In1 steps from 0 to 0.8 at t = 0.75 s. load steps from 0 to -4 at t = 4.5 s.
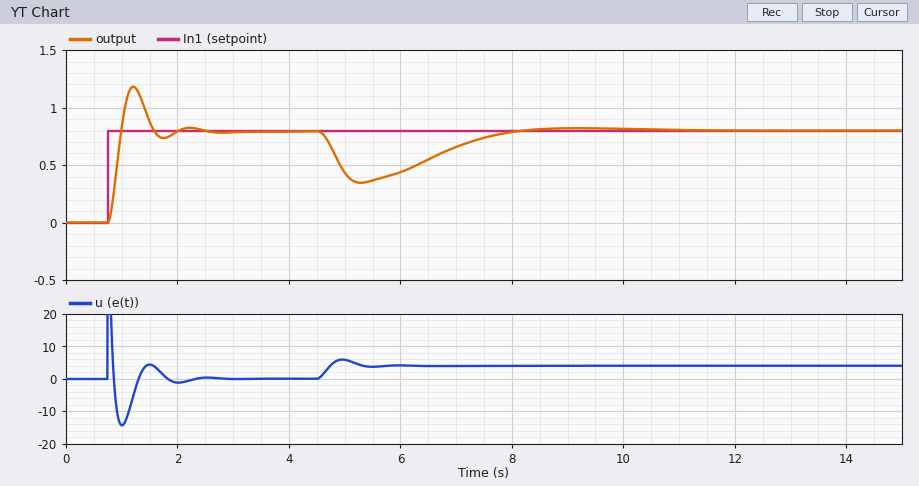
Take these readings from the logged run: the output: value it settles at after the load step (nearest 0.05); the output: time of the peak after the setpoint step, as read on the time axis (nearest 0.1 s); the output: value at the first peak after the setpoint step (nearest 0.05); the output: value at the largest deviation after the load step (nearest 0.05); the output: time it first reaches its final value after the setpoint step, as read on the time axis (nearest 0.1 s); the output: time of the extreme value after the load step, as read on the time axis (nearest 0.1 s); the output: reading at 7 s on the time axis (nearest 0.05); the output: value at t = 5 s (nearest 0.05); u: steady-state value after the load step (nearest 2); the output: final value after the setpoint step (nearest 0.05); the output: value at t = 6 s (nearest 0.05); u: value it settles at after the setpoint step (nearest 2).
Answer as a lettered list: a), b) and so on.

a) 0.80
b) 1.2 s
c) 1.20
d) 0.35
e) 1.0 s
f) 5.3 s
g) 0.65
h) 0.45
i) 4
j) 0.80
k) 0.45
l) 0
